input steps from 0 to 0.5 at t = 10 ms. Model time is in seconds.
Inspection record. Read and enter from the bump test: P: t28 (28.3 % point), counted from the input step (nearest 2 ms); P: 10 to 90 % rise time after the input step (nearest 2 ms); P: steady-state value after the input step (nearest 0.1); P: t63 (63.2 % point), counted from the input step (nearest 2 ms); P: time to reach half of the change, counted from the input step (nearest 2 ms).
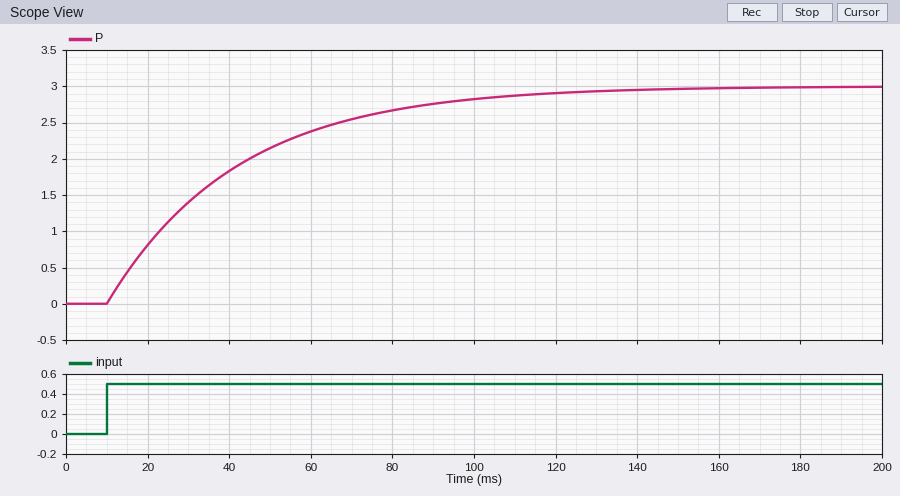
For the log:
10 ms
70 ms
3.0
32 ms
22 ms
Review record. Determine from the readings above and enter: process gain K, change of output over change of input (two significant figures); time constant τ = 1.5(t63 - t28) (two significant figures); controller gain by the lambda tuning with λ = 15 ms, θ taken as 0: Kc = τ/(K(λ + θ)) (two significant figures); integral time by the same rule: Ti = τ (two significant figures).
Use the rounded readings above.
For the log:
6.0
33 ms
0.37
33 ms
